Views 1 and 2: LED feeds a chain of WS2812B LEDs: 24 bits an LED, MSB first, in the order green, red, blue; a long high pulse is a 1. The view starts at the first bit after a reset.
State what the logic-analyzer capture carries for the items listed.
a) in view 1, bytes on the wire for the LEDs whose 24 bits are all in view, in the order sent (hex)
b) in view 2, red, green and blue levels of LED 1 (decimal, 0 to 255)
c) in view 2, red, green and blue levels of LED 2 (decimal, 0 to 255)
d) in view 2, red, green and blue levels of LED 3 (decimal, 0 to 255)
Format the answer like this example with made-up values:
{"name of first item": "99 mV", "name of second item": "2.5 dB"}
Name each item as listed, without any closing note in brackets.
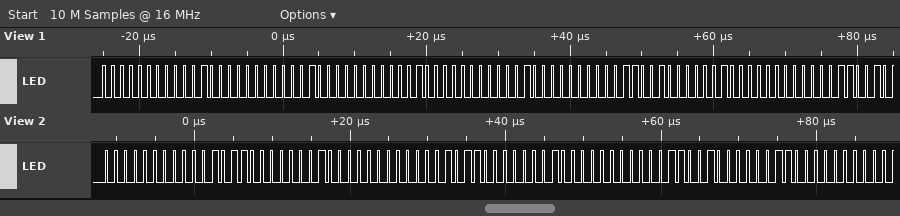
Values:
{"in view 1, bytes on the wire for the LEDs whose 24 bits are all in view, in the order sent": "00 10 01 00 10 01 00 32 04", "in view 2, red, green and blue levels of LED 1": "22, 0, 2", "in view 2, red, green and blue levels of LED 2": "22, 0, 2", "in view 2, red, green and blue levels of LED 3": "50, 0, 6"}
